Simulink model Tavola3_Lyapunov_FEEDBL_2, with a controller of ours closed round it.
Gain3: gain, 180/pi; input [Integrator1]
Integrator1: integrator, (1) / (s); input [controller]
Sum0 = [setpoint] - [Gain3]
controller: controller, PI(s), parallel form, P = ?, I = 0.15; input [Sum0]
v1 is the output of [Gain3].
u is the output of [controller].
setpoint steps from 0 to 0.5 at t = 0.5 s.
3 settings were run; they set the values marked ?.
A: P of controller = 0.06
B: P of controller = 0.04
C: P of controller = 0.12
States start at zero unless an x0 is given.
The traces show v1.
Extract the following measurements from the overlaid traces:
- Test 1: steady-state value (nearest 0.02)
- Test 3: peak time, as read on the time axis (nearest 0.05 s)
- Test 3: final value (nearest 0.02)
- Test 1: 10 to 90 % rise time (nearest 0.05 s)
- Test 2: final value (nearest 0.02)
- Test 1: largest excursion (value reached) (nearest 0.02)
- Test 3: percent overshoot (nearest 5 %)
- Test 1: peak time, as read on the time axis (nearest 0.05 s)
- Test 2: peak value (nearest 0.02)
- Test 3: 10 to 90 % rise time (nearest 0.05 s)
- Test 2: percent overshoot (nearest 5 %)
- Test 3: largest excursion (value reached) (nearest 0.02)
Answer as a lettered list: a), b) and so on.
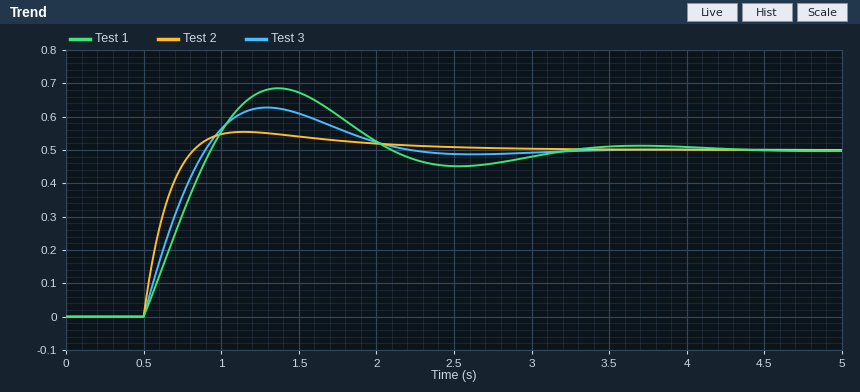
a) 0.50
b) 1.30 s
c) 0.50
d) 0.35 s
e) 0.50
f) 0.68
g) 25 %
h) 1.35 s
i) 0.56
j) 0.30 s
k) 10 %
l) 0.62
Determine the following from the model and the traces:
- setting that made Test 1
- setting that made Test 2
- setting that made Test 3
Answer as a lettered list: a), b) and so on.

a) B
b) C
c) A
